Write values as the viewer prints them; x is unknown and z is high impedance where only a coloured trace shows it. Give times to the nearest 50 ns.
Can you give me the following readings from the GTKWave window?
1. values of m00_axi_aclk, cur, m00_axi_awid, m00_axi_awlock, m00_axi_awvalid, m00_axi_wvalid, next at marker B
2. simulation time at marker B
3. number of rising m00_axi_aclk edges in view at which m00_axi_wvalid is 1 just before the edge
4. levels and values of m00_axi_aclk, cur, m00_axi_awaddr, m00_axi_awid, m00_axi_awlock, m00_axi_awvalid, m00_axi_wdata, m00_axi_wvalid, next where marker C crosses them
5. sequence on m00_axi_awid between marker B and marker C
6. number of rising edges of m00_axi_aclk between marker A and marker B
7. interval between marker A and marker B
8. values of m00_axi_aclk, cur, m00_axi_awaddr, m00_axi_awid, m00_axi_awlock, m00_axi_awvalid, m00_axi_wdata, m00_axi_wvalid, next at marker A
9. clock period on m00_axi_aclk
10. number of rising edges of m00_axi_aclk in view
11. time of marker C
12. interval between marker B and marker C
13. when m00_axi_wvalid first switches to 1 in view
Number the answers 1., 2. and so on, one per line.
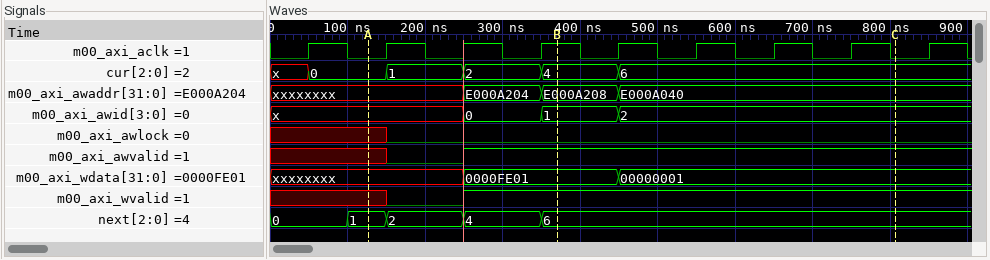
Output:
1. m00_axi_aclk=1, cur=4, m00_axi_awid=1, m00_axi_awlock=0, m00_axi_awvalid=1, m00_axi_wvalid=1, next=6
2. 350 ns
3. 6
4. m00_axi_aclk=0, cur=6, m00_axi_awaddr=E000A040, m00_axi_awid=2, m00_axi_awlock=0, m00_axi_awvalid=1, m00_axi_wdata=00000001, m00_axi_wvalid=1, next=6
5. 1, 2
6. 3
7. 250 ns
8. m00_axi_aclk=0, cur=0, m00_axi_awaddr=xxxxxxxx, m00_axi_awid=x, m00_axi_awlock=x, m00_axi_awvalid=x, m00_axi_wdata=xxxxxxxx, m00_axi_wvalid=x, next=1
9. 100 ns
10. 9
11. 800 ns
12. 450 ns
13. 250 ns
